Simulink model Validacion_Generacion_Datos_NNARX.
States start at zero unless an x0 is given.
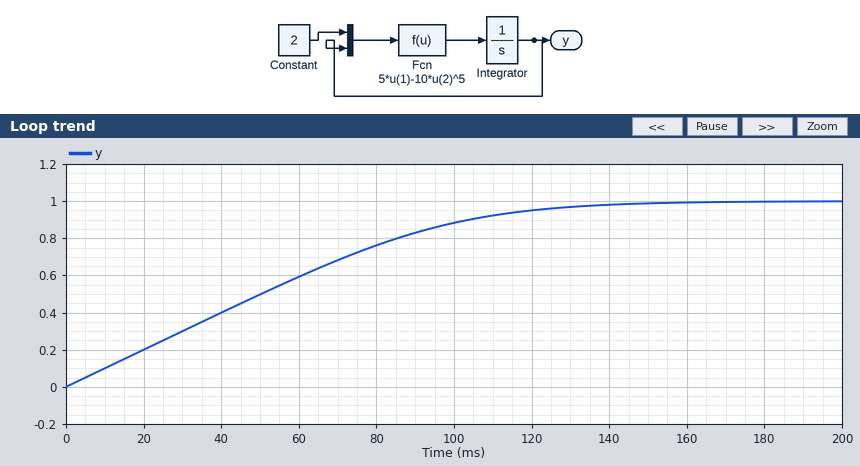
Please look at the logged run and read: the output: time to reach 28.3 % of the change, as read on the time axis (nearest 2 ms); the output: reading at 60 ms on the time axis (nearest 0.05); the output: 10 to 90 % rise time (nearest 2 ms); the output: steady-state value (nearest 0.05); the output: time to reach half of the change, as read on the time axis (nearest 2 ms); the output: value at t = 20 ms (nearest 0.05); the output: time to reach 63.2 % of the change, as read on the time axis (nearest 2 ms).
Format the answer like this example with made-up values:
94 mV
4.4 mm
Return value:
28 ms
0.60
94 ms
1.00
50 ms
0.20
64 ms
